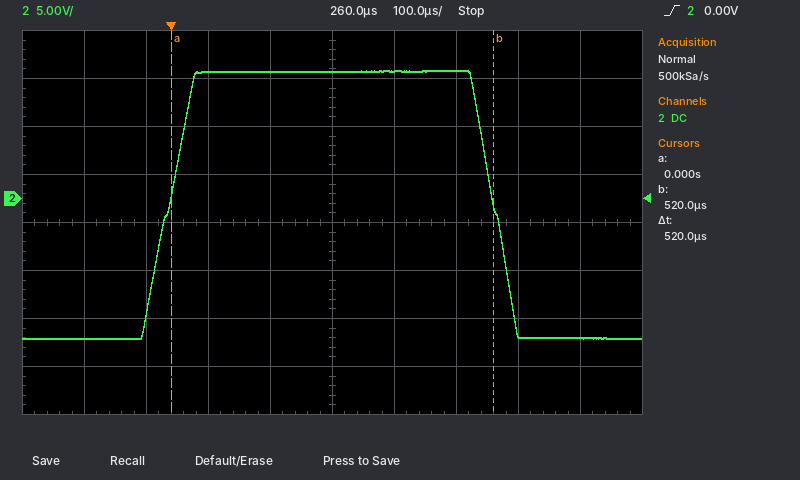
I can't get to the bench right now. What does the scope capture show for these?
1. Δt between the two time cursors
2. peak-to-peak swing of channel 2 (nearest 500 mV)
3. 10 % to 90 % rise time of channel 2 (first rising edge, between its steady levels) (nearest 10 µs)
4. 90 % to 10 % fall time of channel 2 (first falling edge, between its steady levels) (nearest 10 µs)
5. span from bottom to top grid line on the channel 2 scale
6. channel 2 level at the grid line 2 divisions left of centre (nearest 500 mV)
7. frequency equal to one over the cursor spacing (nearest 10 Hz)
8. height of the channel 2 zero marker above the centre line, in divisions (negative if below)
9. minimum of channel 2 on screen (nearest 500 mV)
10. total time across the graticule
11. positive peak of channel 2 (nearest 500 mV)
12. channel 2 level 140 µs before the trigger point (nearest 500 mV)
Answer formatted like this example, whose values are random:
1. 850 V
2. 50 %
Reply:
1. 520 µs
2. 28.0 V
3. 70 µs
4. 60 µs
5. 40 V
6. 13.0 V
7. 1.92 kHz
8. +0.5 div
9. -14.5 V
10. 1 ms
11. 13.5 V
12. -14.5 V
